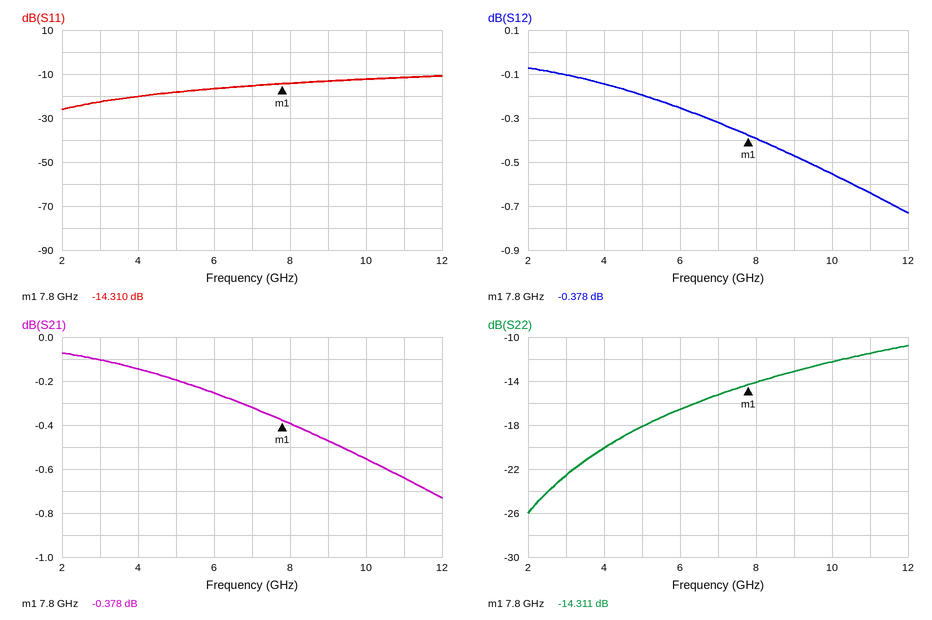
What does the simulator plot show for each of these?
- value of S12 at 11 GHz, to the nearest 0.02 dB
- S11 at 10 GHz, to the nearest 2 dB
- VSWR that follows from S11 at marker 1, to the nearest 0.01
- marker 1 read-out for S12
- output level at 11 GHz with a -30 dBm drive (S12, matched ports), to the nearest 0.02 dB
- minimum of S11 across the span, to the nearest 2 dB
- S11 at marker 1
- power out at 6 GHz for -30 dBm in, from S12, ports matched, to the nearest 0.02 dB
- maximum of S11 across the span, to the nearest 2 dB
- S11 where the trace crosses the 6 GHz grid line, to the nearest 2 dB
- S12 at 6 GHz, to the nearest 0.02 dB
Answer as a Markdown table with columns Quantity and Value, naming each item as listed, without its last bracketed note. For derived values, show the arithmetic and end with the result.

| Quantity | Value |
|---|---|
| value of S12 at 11 GHz, to the nearest 0.02 dB | -0.64 dB |
| S11 at 10 GHz, to the nearest 2 dB | -12 dB |
| VSWR that follows from S11 at marker 1, to the nearest 0.01 | (1 + 0.1925)/(1 − 0.1925) ≈ 1.48 |
| marker 1 read-out for S12 | -0.378 dB |
| output level at 11 GHz with a -30 dBm drive (S12, matched ports), to the nearest 0.02 dB | -30 dBm + (-0.64 dB) = -30.64 dBm |
| minimum of S11 across the span, to the nearest 2 dB | -26 dB |
| S11 at marker 1 | -14.310 dB |
| power out at 6 GHz for -30 dBm in, from S12, ports matched, to the nearest 0.02 dB | -30 dBm + (-0.26 dB) = -30.26 dBm |
| maximum of S11 across the span, to the nearest 2 dB | -10 dB |
| S11 where the trace crosses the 6 GHz grid line, to the nearest 2 dB | -16 dB |
| S12 at 6 GHz, to the nearest 0.02 dB | -0.26 dB |
